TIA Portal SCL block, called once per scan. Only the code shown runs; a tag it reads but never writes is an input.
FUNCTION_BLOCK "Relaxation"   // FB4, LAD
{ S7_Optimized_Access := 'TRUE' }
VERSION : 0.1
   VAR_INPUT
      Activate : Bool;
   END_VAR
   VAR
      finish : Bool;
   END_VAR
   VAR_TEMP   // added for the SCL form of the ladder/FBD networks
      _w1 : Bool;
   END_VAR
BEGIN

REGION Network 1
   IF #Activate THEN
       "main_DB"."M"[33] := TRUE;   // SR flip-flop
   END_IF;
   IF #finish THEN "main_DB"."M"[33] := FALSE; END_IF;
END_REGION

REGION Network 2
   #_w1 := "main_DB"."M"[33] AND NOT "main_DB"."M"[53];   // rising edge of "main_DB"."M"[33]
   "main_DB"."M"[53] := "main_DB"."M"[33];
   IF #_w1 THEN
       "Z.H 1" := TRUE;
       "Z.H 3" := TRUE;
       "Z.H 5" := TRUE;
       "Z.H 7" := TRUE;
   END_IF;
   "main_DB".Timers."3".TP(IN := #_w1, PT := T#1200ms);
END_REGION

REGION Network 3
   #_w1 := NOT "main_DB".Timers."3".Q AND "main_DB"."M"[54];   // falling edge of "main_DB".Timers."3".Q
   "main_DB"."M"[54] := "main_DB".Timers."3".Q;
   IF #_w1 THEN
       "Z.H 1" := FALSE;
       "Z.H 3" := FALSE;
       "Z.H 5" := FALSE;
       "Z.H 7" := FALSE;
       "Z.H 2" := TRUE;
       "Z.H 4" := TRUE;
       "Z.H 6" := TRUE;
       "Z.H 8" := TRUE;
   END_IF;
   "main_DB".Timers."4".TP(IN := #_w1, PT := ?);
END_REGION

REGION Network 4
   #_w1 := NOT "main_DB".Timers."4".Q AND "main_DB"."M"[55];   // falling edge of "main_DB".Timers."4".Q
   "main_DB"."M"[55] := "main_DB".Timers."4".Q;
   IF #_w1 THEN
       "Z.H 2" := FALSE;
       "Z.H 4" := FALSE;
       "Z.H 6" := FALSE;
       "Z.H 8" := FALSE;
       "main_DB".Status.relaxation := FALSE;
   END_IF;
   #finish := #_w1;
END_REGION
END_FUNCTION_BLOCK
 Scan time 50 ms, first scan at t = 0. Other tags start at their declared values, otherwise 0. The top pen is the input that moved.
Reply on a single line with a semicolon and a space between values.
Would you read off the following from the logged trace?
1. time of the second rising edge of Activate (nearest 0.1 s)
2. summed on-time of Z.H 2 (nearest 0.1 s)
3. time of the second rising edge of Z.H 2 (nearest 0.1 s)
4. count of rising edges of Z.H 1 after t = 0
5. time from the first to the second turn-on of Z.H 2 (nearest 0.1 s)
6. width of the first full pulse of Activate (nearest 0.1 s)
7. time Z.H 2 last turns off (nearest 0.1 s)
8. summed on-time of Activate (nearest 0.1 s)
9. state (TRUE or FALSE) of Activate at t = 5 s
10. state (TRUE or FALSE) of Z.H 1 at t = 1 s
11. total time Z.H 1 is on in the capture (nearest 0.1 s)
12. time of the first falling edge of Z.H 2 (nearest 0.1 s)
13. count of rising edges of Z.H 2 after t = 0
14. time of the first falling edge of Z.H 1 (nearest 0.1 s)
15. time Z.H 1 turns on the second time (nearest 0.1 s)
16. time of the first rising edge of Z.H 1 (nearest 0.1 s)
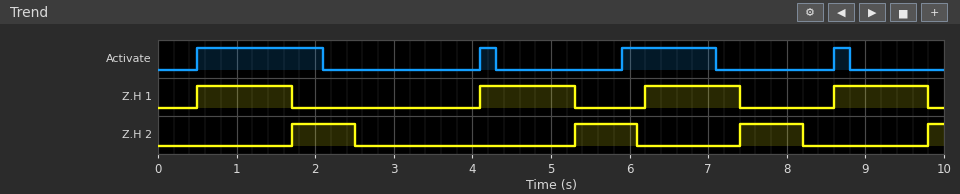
4.1 s; 2.6 s; 5.3 s; 4; 3.6 s; 1.6 s; 8.2 s; 3.2 s; FALSE; TRUE; 4.8 s; 2.5 s; 4; 1.7 s; 4.1 s; 0.5 s
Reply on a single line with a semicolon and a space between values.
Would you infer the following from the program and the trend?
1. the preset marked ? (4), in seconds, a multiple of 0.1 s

0.8 s
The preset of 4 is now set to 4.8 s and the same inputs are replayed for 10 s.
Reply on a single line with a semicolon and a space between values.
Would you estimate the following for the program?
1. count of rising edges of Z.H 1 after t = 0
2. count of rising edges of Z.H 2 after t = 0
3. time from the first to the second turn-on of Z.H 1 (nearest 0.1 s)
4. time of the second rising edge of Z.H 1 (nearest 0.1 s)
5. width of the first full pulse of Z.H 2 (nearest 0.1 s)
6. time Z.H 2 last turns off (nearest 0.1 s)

2; 2; 6.1 s; 6.6 s; 4.8 s; 6.5 s
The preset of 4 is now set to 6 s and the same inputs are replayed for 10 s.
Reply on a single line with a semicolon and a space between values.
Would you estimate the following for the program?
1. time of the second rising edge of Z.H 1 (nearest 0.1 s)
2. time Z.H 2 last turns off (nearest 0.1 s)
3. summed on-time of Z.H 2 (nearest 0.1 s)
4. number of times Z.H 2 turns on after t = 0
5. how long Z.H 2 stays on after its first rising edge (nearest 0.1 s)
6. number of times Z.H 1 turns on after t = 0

8.6 s; 7.7 s; 6.2 s; 2; 6.0 s; 2
